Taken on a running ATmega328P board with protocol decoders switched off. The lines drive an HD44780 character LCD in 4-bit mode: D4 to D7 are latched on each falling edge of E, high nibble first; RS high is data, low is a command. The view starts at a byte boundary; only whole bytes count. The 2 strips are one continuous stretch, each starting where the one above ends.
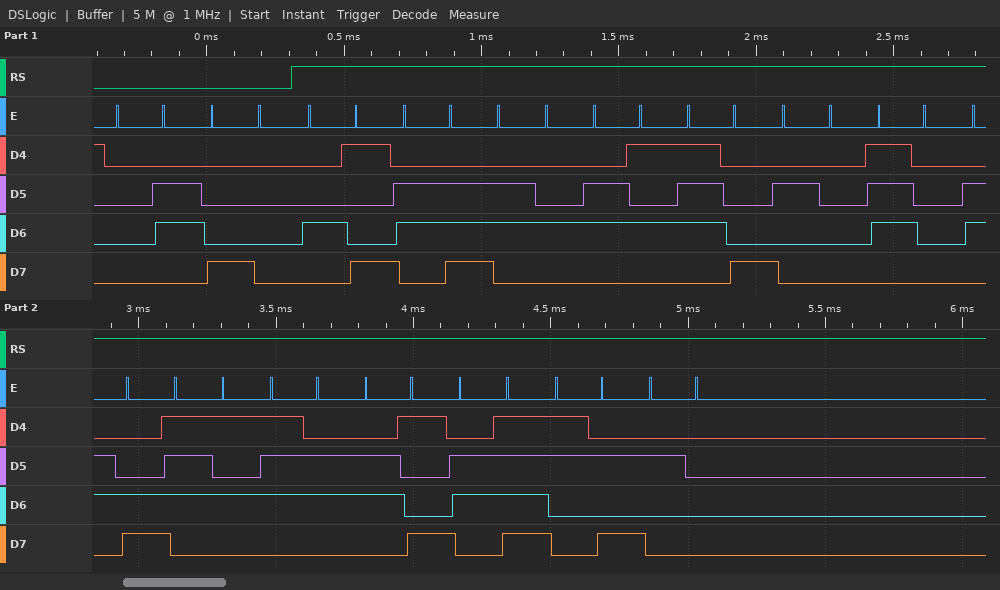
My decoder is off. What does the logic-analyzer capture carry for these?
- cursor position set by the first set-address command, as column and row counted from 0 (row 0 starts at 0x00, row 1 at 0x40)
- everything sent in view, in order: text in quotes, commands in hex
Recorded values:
column 0, row 0
0x06 0x80 "Index pluvio: "
